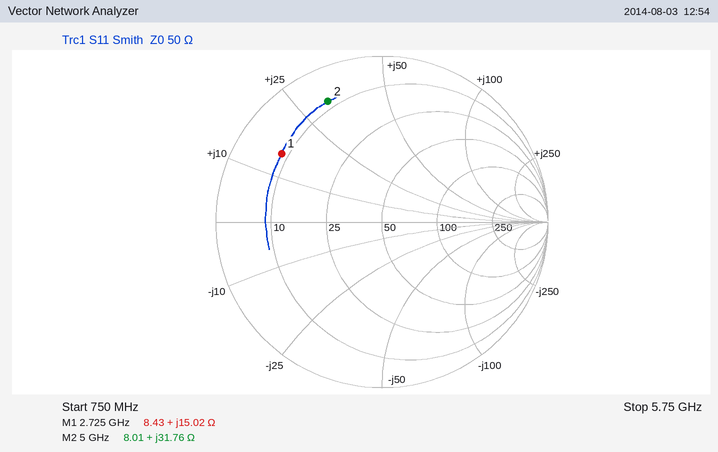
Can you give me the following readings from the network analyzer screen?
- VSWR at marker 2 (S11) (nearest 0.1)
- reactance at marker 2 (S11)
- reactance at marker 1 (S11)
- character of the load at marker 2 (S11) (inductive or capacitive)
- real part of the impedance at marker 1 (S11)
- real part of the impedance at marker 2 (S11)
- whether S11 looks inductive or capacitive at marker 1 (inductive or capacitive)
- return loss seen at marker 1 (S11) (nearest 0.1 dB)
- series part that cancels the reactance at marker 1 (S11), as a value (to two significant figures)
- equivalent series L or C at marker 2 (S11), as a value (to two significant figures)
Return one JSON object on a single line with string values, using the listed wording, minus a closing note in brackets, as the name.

{"VSWR at marker 2 (S11)": "8.8", "reactance at marker 2": "+31.76 Ω", "reactance at marker 1": "+15.02 Ω", "character of the load at marker 2 (S11)": "inductive", "real part of the impedance at marker 1": "8.43 Ω", "real part of the impedance at marker 2": "8.01 Ω", "whether S11 looks inductive or capacitive at marker 1": "inductive", "return loss seen at marker 1 (S11)": "2.7 dB", "series part that cancels the reactance at marker 1 (S11), as a value": "3.9 pF", "equivalent series L or C at marker 2 (S11), as a value": "1.0 nH"}
